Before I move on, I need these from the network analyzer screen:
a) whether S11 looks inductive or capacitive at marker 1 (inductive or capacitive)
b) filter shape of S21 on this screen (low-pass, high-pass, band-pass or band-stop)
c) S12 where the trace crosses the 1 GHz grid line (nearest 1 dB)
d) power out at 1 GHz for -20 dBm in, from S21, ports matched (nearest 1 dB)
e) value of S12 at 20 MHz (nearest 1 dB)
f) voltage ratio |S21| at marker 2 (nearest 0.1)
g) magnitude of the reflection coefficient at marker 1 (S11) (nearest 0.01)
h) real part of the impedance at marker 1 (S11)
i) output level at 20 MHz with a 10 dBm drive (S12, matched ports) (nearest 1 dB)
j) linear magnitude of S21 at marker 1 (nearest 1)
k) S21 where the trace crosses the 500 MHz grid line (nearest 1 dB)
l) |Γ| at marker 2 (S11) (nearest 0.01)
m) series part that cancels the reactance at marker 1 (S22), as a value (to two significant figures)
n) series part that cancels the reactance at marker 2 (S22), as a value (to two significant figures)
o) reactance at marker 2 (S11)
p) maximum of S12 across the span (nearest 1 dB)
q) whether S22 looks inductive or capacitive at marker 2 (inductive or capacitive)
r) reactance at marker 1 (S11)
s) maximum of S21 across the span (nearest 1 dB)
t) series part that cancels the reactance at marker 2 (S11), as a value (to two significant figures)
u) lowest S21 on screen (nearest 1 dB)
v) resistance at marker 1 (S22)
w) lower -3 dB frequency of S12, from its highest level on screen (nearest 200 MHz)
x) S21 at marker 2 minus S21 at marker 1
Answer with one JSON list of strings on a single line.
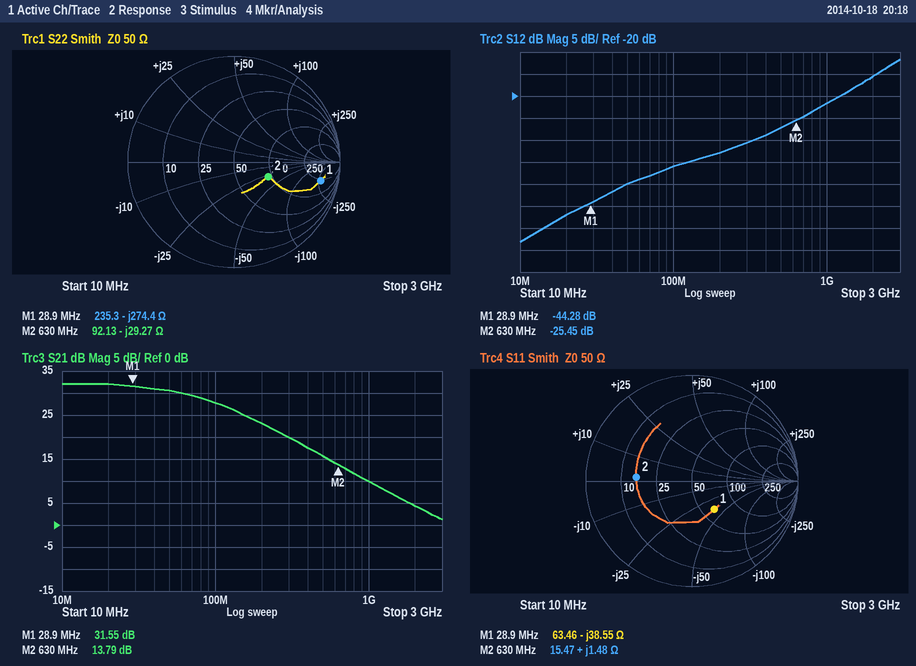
["capacitive", "low-pass", "-22 dB", "-10 dBm", "-47 dB", "4.9", "0.34", "63.46 Ω", "-37 dBm", "38", "16 dB", "0.53", "1.5 µH", "7.4 nH", "+1.48 Ω", "-12 dB", "capacitive", "-38.55 Ω", "32 dB", "170 pF", "1 dB", "235.3 Ω", "2.2 GHz", "-17.76 dB"]
